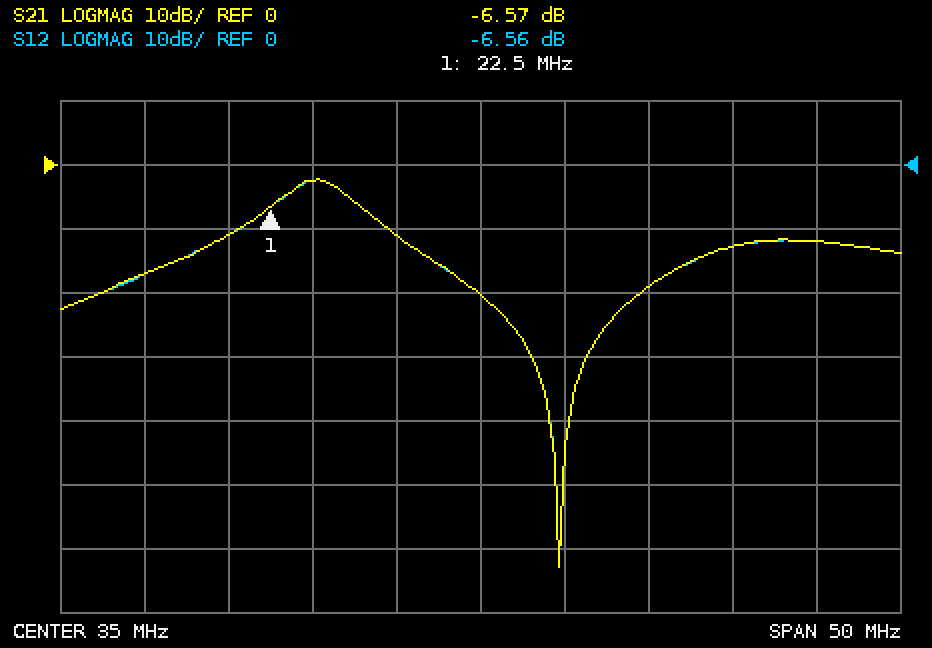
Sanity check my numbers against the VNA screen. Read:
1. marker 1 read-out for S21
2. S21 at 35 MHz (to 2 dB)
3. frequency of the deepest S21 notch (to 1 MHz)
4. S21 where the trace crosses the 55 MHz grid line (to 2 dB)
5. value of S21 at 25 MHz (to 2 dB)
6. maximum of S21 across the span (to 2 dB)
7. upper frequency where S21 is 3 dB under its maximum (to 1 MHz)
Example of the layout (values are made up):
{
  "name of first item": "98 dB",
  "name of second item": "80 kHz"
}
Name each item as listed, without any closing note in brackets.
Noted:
{
  "marker 1 read-out for S21": "-6.57 dB",
  "S21 at 35 MHz": "-20 dB",
  "frequency of the deepest S21 notch": "40 MHz",
  "S21 where the trace crosses the 55 MHz grid line": "-12 dB",
  "value of S21 at 25 MHz": "-2 dB",
  "maximum of S21 across the span": "-2 dB",
  "upper frequency where S21 is 3 dB under its maximum": "27 MHz"
}
